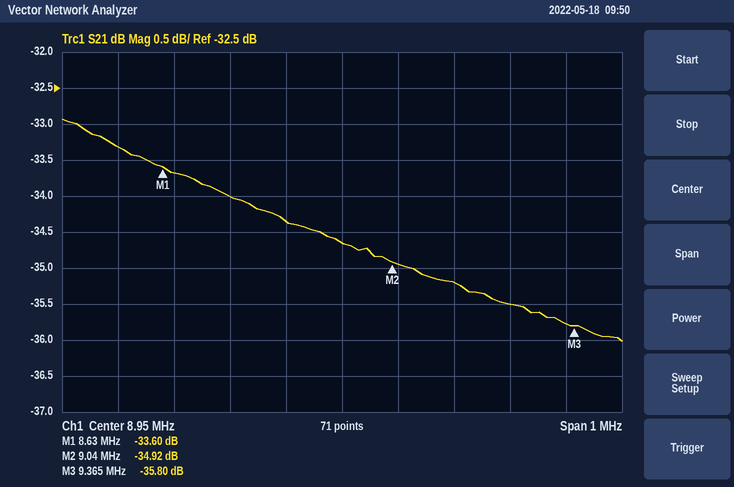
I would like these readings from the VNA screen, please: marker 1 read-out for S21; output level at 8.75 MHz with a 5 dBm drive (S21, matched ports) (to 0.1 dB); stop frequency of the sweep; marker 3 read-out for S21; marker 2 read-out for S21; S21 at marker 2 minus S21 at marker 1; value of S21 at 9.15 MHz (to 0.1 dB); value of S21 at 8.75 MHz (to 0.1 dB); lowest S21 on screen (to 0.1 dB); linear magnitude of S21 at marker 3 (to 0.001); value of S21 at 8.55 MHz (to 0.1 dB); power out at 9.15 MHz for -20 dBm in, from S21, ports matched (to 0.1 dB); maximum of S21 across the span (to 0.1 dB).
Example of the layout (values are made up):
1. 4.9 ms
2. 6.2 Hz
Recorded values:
1. -33.60 dB
2. -29.0 dBm
3. 9.45 MHz
4. -35.80 dB
5. -34.92 dB
6. -1.32 dB
7. -35.2 dB
8. -34.0 dB
9. -36.0 dB
10. 0.016
11. -33.3 dB
12. -55.2 dBm
13. -32.9 dB
